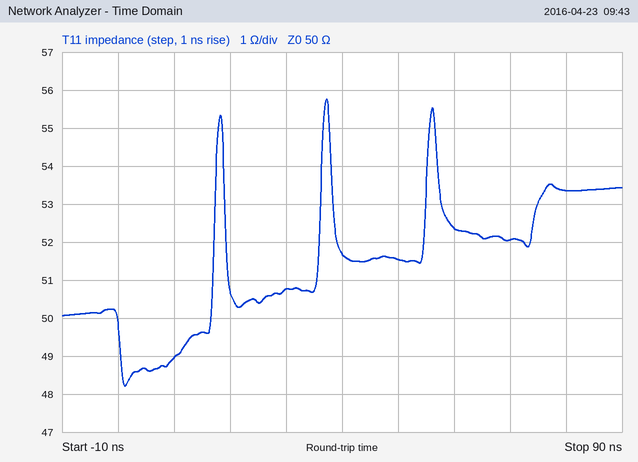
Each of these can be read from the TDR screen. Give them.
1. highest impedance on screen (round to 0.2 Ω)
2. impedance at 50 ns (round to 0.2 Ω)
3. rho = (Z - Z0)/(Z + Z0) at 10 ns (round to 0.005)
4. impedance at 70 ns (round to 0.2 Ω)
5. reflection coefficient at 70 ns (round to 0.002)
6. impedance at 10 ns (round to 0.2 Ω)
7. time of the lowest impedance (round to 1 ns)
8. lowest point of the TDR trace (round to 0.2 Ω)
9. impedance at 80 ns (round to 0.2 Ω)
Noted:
55.8 Ω
51.6 Ω
-0.010
52.0 Ω
+0.020
49.0 Ω
1 ns
48.2 Ω
53.4 Ω
